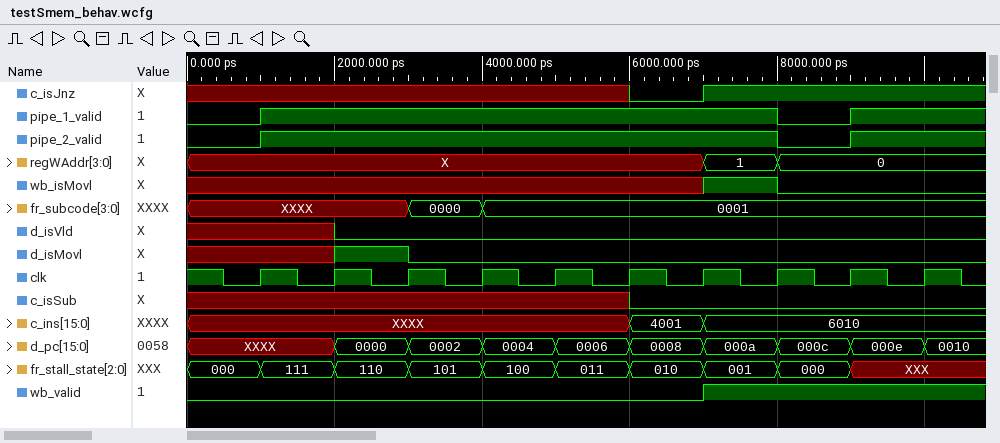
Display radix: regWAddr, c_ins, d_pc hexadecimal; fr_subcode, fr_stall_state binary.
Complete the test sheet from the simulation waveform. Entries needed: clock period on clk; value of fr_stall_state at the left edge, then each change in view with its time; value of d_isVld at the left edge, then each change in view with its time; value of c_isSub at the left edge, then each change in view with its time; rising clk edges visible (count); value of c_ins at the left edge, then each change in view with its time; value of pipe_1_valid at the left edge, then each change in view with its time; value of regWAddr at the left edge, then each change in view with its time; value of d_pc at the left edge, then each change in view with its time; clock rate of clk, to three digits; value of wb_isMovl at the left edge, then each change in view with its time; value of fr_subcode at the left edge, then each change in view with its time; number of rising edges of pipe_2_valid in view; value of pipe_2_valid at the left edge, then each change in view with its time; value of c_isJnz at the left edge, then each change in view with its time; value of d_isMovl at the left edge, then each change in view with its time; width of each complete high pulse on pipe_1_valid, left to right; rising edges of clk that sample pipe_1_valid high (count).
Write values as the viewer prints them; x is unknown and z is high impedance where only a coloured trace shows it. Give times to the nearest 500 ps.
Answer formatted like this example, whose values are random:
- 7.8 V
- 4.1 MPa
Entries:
- 1000 ps
- 000, 111 at 1000 ps, 110 at 2000 ps, 101 at 3000 ps, 100 at 4000 ps, 011 at 5000 ps, 010 at 6000 ps, 001 at 7000 ps, 000 at 8000 ps, XXX at 9000 ps
- x, 0 at 2000 ps
- x, 0 at 6000 ps
- 10
- XXXX, 4001 at 6000 ps, 6010 at 7000 ps
- 0, 1 at 1000 ps, 0 at 8000 ps, 1 at 9000 ps
- X, 1 at 7000 ps, 0 at 8000 ps
- XXXX, 0000 at 2000 ps, 0002 at 3000 ps, 0004 at 4000 ps, 0006 at 5000 ps, 0008 at 6000 ps, 000a at 7000 ps, 000c at 8000 ps, 000e at 9000 ps, 0010 at 10000 ps
- 1.00 GHz
- x, 1 at 7000 ps, 0 at 8000 ps
- XXXX, 0000 at 3000 ps, 0001 at 4000 ps
- 2
- 0, 1 at 1000 ps, 0 at 8000 ps, 1 at 9000 ps
- x, 0 at 6000 ps, 1 at 7000 ps
- x, 1 at 2000 ps, 0 at 3000 ps
- 7000 ps
- 8
